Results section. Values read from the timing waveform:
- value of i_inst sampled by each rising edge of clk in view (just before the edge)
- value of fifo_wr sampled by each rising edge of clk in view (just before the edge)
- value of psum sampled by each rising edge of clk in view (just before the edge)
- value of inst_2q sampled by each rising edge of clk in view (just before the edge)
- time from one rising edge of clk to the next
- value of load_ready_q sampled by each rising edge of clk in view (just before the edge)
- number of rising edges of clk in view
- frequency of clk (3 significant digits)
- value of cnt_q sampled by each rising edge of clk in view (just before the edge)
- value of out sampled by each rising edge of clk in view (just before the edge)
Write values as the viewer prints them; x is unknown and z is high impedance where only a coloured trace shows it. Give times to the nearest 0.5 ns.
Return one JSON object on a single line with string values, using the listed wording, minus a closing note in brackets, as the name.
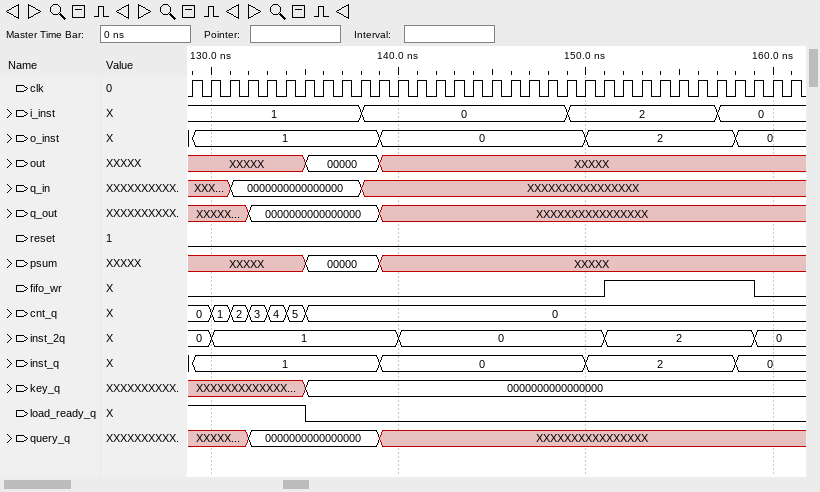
{"value of i_inst sampled by each rising edge of clk in view": "1, 1, 1, 1, 1, 1, 1, 1, 1, 1, 0, 0, 0, 0, 0, 0, 0, 0, 0, 0, 0, 2, 2, 2, 2, 2, 2, 2, 2, 0, 0, 0, 0", "value of fifo_wr sampled by each rising edge of clk in view": "0 0 0 0 0 0 0 0 0 0 0 0 0 0 0 0 0 0 0 0 0 0 0 1 1 1 1 1 1 1 1 0 0", "value of psum sampled by each rising edge of clk in view": "XXXXX, XXXXX, XXXXX, XXXXX, XXXXX, XXXXX, XXXXX, 00000, 00000, 00000, 00000, XXXXX, XXXXX, XXXXX, XXXXX, XXXXX, XXXXX, XXXXX, XXXXX, XXXXX, XXXXX, XXXXX, XXXXX, XXXXX, XXXXX, XXXXX, XXXXX, XXXXX, XXXXX, XXXXX, XXXXX, XXXXX, XXXXX", "value of inst_2q sampled by each rising edge of clk in view": "0, 0, 1, 1, 1, 1, 1, 1, 1, 1, 1, 1, 0, 0, 0, 0, 0, 0, 0, 0, 0, 0, 0, 2, 2, 2, 2, 2, 2, 2, 2, 0, 0", "time from one rising edge of clk to the next": "1 ns", "value of load_ready_q sampled by each rising edge of clk in view": "1 1 1 1 1 1 1 0 0 0 0 0 0 0 0 0 0 0 0 0 0 0 0 0 0 0 0 0 0 0 0 0 0", "number of rising edges of clk in view": "33", "frequency of clk": "1.00 GHz", "value of cnt_q sampled by each rising edge of clk in view": "0, 0, 1, 2, 3, 4, 5, 0, 0, 0, 0, 0, 0, 0, 0, 0, 0, 0, 0, 0, 0, 0, 0, 0, 0, 0, 0, 0, 0, 0, 0, 0, 0", "value of out sampled by each rising edge of clk in view": "XXXXX, XXXXX, XXXXX, XXXXX, XXXXX, XXXXX, XXXXX, 00000, 00000, 00000, 00000, XXXXX, XXXXX, XXXXX, XXXXX, XXXXX, XXXXX, XXXXX, XXXXX, XXXXX, XXXXX, XXXXX, XXXXX, XXXXX, XXXXX, XXXXX, XXXXX, XXXXX, XXXXX, XXXXX, XXXXX, XXXXX, XXXXX"}
